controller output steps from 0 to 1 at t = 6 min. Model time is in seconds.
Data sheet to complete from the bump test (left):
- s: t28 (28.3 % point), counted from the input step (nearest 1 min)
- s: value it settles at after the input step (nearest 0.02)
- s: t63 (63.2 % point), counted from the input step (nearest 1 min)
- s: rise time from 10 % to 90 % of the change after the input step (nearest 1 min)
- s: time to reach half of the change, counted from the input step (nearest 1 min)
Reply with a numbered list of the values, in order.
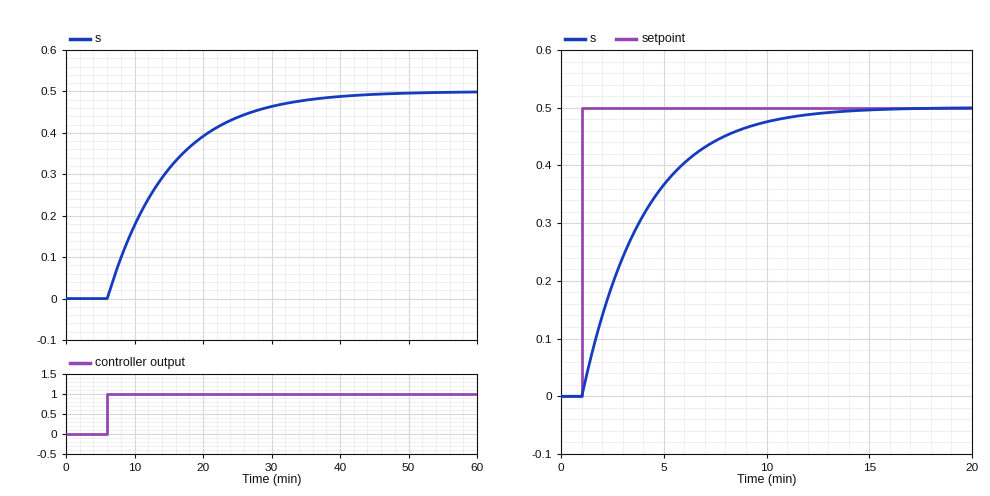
1. 3 min
2. 0.50
3. 9 min
4. 20 min
5. 6 min
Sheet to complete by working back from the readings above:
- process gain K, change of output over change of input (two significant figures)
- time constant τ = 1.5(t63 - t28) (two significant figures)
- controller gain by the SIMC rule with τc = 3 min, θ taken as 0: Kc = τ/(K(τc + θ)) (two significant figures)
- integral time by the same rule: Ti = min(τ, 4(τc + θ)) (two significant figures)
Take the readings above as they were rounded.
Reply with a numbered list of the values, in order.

1. 0.50
2. 9.0 min
3. 6.0
4. 9.0 min
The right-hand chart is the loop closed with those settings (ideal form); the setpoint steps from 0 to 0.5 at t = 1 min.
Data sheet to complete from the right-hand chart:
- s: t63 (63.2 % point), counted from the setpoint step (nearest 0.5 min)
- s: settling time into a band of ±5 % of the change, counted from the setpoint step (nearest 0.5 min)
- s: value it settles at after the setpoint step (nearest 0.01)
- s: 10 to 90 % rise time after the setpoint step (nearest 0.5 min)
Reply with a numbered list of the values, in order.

1. 3.0 min
2. 9.0 min
3. 0.50
4. 6.5 min
